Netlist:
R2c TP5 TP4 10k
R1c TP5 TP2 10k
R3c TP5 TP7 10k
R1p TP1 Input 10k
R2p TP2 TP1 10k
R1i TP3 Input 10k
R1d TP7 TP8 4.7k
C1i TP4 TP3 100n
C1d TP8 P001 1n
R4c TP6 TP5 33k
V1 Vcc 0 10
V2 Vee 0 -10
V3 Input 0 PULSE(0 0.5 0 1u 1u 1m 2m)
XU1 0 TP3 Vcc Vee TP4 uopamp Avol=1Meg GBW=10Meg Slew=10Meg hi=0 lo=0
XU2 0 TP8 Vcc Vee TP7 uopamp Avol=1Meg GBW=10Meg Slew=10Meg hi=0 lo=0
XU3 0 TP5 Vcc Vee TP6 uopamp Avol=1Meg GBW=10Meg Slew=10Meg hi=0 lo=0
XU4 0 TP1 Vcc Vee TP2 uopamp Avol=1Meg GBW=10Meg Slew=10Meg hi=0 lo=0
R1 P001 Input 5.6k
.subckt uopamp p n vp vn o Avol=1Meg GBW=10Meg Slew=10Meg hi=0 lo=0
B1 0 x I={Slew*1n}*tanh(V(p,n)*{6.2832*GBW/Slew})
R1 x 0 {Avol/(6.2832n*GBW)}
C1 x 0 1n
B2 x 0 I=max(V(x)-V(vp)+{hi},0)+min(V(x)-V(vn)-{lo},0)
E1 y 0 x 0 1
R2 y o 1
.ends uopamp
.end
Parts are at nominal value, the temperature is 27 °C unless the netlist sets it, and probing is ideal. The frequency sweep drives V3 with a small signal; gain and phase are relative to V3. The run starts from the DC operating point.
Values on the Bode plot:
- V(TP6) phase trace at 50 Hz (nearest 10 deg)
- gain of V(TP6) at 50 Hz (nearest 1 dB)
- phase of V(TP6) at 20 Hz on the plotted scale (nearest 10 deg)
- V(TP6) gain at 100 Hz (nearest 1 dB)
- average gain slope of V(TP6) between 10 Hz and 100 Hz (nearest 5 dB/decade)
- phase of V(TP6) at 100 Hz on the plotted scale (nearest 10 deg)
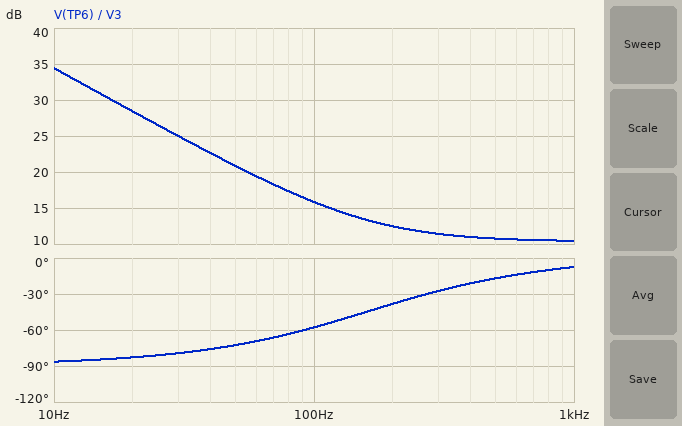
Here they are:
-70 deg
21 dB
-80 deg
16 dB
-20 dB/decade
-60 deg
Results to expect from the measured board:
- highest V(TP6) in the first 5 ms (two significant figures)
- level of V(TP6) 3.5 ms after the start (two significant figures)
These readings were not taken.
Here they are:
6.6 V
3.3 V
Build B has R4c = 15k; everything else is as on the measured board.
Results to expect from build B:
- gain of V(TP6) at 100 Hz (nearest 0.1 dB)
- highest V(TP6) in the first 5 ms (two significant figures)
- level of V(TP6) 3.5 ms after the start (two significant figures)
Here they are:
9.0 dB
3.0 V
1.5 V
